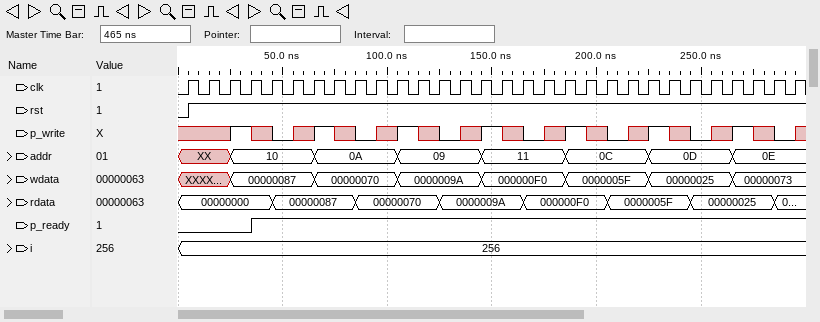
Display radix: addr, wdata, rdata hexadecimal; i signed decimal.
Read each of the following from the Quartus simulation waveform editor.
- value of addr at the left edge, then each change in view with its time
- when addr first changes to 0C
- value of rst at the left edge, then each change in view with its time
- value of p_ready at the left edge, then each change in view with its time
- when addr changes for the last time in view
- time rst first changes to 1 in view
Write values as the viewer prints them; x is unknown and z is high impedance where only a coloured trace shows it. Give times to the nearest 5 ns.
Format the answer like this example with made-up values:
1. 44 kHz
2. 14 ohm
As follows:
1. XX, 10 at 25 ns, 0A at 65 ns, 09 at 105 ns, 11 at 145 ns, 0C at 185 ns, 0D at 225 ns, 0E at 265 ns
2. 185 ns
3. 0, 1 at 5 ns
4. 0, 1 at 35 ns
5. 265 ns
6. 5 ns
